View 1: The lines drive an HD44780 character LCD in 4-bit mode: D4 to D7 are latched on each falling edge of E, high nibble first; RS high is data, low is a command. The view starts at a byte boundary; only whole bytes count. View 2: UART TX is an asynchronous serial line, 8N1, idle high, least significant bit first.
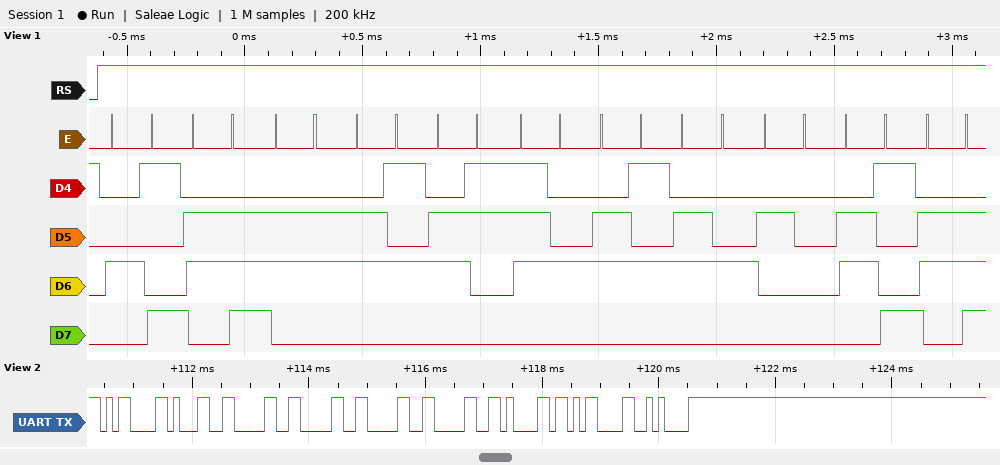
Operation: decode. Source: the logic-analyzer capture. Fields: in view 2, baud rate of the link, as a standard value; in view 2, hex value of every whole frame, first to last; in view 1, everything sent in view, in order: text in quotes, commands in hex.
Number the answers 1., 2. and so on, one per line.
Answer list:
1. 9600 baud
2. 0D 31 30 30 30 30 61 0D 0A
3. "Infected in"
